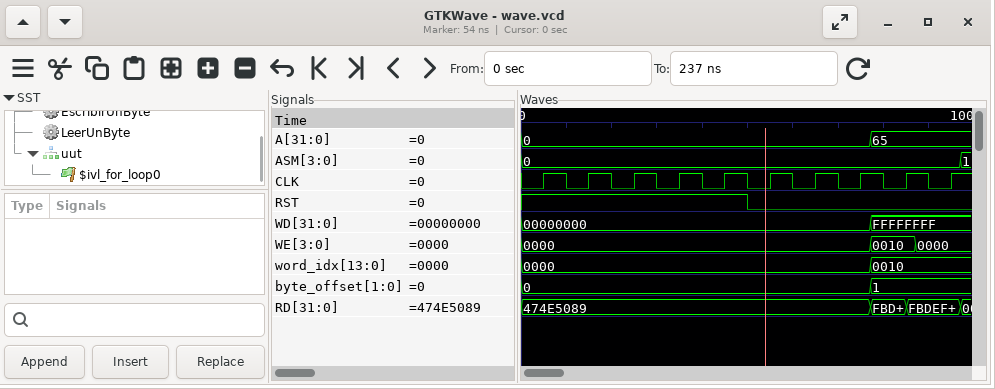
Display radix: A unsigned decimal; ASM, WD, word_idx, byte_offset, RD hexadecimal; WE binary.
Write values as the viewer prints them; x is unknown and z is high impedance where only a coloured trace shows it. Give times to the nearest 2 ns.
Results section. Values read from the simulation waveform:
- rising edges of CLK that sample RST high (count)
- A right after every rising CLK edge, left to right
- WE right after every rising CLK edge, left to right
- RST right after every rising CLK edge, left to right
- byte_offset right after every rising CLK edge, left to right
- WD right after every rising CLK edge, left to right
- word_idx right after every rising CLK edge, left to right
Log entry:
5
0, 0, 0, 0, 0, 0, 0, 0, 65, 65
0000, 0000, 0000, 0000, 0000, 0000, 0000, 0000, 0010, 0000
1 1 1 1 1 0 0 0 0 0
0, 0, 0, 0, 0, 0, 0, 0, 1, 1
00000000, 00000000, 00000000, 00000000, 00000000, 00000000, 00000000, 00000000, FFFFFFFF, FFFFFFFF
0000, 0000, 0000, 0000, 0000, 0000, 0000, 0000, 0010, 0010
